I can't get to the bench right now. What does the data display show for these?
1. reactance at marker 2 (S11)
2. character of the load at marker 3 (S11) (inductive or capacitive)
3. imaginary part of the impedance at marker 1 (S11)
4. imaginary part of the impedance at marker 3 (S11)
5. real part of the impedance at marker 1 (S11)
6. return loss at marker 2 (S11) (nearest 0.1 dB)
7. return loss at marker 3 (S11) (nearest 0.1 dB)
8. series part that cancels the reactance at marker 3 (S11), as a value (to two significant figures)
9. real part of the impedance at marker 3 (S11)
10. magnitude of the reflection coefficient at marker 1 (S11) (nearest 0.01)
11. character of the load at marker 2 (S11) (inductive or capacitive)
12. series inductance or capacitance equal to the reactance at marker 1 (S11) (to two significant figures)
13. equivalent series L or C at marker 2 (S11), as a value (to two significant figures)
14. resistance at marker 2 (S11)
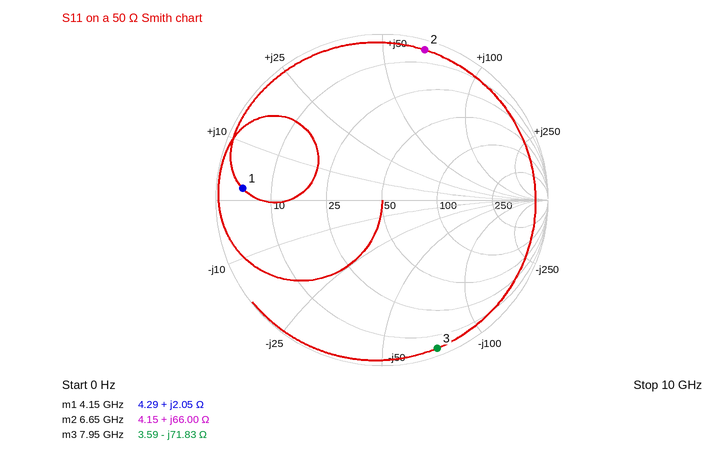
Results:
+66.00 Ω
capacitive
+2.05 Ω
-71.83 Ω
4.29 Ω
0.5 dB
0.4 dB
1.4 nH
3.59 Ω
0.84
inductive
79 pH
1.6 nH
4.15 Ω
